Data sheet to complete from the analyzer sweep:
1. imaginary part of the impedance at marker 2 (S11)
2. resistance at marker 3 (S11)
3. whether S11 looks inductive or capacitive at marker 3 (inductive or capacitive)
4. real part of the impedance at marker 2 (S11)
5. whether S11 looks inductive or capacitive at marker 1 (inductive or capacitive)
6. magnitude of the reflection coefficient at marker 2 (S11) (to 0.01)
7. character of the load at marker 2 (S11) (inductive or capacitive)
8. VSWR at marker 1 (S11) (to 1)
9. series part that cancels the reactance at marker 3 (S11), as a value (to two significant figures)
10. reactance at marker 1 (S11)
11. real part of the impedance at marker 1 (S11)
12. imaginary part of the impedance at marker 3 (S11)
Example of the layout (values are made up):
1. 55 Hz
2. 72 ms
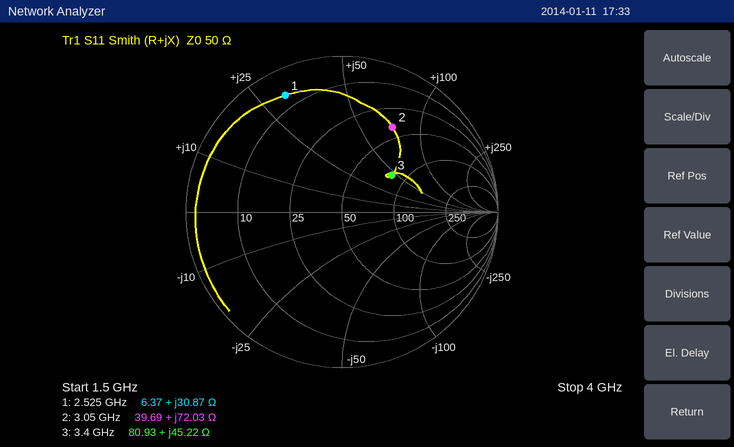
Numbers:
1. +72.03 Ω
2. 80.93 Ω
3. inductive
4. 39.69 Ω
5. inductive
6. 0.63
7. inductive
8. 11
9. 1.0 pF
10. +30.87 Ω
11. 6.37 Ω
12. +45.22 Ω
